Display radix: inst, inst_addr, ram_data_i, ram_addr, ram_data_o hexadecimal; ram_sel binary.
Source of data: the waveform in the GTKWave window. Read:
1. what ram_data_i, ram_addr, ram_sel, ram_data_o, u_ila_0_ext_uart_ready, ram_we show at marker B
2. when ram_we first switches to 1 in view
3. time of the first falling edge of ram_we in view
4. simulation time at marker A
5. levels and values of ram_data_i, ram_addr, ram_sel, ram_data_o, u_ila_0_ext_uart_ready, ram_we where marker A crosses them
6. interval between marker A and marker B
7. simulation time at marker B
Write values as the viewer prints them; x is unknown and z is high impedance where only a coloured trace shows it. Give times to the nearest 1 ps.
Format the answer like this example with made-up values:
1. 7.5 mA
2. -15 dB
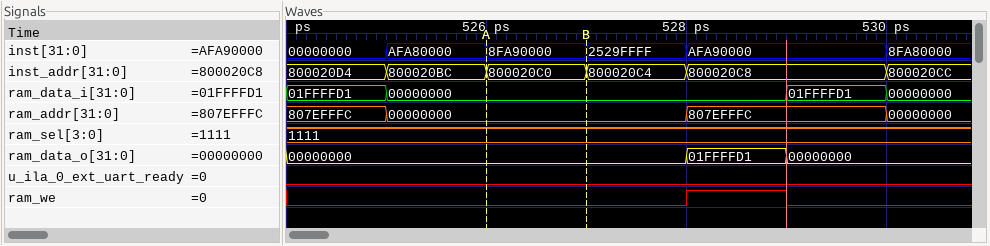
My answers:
1. ram_data_i=00000000, ram_addr=00000000, ram_sel=1111, ram_data_o=00000000, u_ila_0_ext_uart_ready=0, ram_we=0
2. 528 ps
3. 529 ps
4. 526 ps
5. ram_data_i=00000000, ram_addr=00000000, ram_sel=1111, ram_data_o=00000000, u_ila_0_ext_uart_ready=0, ram_we=0
6. 1 ps
7. 527 ps
